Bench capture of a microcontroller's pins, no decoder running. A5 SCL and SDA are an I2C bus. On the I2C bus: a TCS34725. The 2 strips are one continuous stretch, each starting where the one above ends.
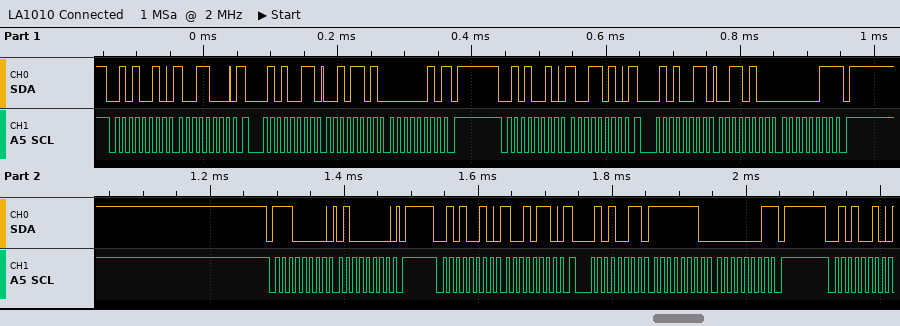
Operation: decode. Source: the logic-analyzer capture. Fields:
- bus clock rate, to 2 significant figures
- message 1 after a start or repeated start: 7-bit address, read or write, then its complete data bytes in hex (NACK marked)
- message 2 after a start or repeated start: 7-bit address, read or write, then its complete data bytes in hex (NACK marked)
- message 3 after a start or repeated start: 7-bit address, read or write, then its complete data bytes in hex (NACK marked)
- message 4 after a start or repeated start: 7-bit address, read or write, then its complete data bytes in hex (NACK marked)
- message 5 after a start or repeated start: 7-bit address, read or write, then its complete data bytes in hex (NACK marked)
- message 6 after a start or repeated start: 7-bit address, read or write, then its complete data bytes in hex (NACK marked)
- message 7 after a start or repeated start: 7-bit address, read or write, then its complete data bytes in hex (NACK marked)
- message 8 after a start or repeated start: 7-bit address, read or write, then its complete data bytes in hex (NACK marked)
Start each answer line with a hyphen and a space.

- 100 kHz
- 0x29 write: 98
- 0x29 read: 2D 02 NACK
- 0x29 write: 9A
- 0x29 read: 34 03 NACK
- 0x70 write: 40
- 0x29 write: 96
- 0x29 read: FE 01 NACK
- 0x29 write
